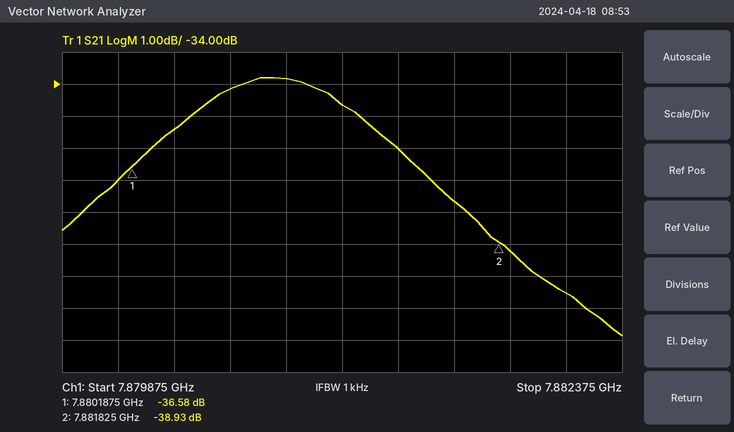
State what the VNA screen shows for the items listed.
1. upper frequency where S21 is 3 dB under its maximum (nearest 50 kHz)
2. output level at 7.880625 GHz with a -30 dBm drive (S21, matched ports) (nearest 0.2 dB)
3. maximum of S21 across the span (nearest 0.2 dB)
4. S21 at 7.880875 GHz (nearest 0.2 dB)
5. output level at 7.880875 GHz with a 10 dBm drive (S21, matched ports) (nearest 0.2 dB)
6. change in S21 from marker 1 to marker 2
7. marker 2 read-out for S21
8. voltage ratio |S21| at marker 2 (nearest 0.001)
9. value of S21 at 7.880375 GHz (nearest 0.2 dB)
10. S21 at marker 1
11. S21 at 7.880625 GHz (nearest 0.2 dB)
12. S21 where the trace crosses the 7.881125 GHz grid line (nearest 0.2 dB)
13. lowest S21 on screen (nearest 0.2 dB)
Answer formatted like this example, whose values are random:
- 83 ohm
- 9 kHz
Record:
- 7.88150 GHz
- -64.2 dBm
- -33.8 dB
- -33.8 dB
- -23.8 dBm
- -2.35 dB
- -38.93 dB
- 0.011
- -35.4 dB
- -36.58 dB
- -34.2 dB
- -34.6 dB
- -41.8 dB
